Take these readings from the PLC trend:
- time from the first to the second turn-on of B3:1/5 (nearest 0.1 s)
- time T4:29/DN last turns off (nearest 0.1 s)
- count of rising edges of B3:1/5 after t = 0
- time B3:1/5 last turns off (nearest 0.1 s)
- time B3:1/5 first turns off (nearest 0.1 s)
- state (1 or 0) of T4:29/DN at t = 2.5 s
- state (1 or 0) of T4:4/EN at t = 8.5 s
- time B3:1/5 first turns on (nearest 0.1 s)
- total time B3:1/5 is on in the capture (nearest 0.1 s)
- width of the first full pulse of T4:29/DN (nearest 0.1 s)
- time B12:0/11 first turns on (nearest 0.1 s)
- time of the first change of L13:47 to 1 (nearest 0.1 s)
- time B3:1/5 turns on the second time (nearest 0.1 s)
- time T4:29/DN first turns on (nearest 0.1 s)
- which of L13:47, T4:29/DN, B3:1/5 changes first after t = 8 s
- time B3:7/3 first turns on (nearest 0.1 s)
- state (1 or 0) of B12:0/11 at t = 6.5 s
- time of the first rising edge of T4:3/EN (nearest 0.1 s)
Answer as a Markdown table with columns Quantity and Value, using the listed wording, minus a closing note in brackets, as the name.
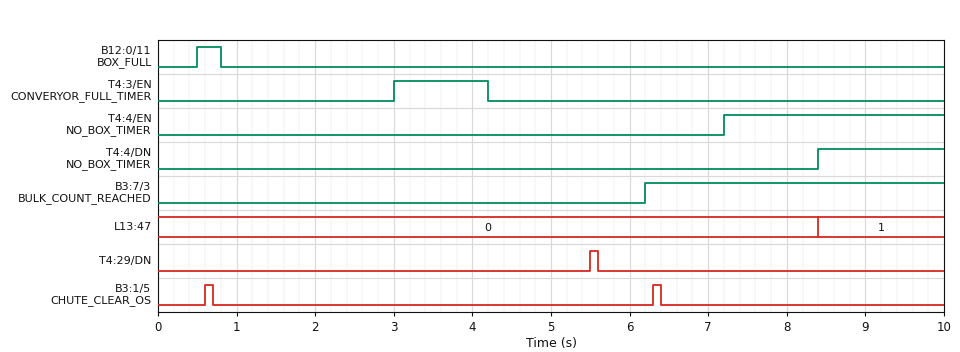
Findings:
| Quantity | Value |
|---|---|
| time from the first to the second turn-on of B3:1/5 | 5.7 s |
| time T4:29/DN last turns off | 5.6 s |
| count of rising edges of B3:1/5 after t = 0 | 2 |
| time B3:1/5 last turns off | 6.4 s |
| time B3:1/5 first turns off | 0.7 s |
| state (1 or 0) of T4:29/DN at t = 2.5 s | 0 |
| state (1 or 0) of T4:4/EN at t = 8.5 s | 1 |
| time B3:1/5 first turns on | 0.6 s |
| total time B3:1/5 is on in the capture | 0.2 s |
| width of the first full pulse of T4:29/DN | 0.1 s |
| time B12:0/11 first turns on | 0.5 s |
| time of the first change of L13:47 to 1 | 8.4 s |
| time B3:1/5 turns on the second time | 6.3 s |
| time T4:29/DN first turns on | 5.5 s |
| which of L13:47, T4:29/DN, B3:1/5 changes first after t = 8 s | L13:47 |
| time B3:7/3 first turns on | 6.2 s |
| state (1 or 0) of B12:0/11 at t = 6.5 s | 0 |
| time of the first rising edge of T4:3/EN | 3.0 s |
